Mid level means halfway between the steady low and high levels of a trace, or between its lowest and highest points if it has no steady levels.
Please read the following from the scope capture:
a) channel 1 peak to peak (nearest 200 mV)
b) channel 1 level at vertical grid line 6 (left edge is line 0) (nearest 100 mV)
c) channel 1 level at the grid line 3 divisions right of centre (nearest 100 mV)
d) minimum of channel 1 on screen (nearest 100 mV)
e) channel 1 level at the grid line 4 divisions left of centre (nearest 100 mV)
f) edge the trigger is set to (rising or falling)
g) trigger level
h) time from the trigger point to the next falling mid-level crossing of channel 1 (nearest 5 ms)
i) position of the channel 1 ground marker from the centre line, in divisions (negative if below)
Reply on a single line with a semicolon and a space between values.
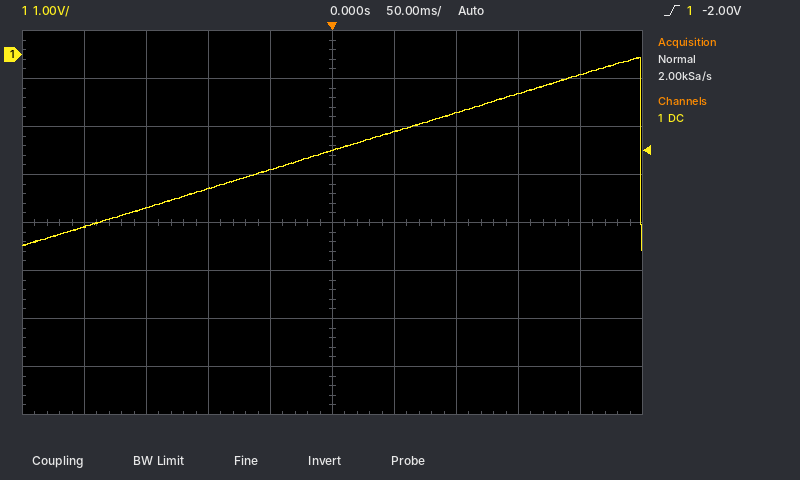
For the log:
4.0 V; -1.6 V; -800 mV; -4.1 V; -3.6 V; rising; -2.00 V; 250 ms; +3.5 div
